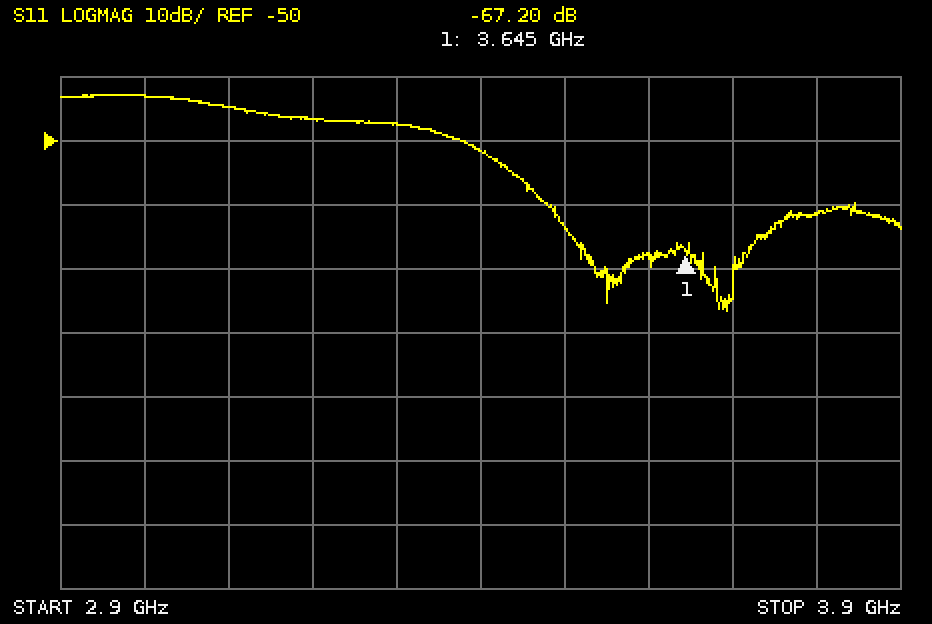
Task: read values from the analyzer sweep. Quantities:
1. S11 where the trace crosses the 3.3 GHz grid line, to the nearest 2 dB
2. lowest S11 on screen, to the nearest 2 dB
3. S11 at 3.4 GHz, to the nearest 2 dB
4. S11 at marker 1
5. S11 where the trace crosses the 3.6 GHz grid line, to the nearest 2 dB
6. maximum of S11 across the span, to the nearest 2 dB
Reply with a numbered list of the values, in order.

1. -48 dB
2. -76 dB
3. -52 dB
4. -67.20 dB
5. -68 dB
6. -42 dB
